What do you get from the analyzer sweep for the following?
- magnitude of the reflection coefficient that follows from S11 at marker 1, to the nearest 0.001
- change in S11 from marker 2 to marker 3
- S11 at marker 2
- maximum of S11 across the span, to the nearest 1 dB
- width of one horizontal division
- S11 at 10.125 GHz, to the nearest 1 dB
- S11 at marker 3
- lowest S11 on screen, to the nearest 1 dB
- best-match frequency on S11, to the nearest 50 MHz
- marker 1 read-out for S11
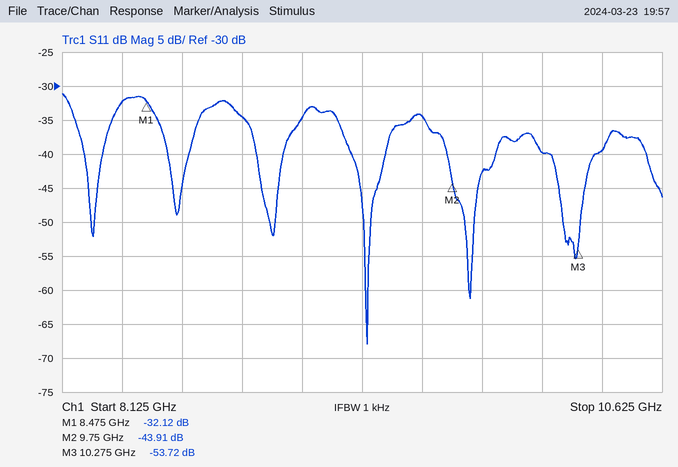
0.025
-9.81 dB
-43.91 dB
-31 dB
250 MHz
-40 dB
-53.72 dB
-68 dB
9.40 GHz
-32.12 dB
